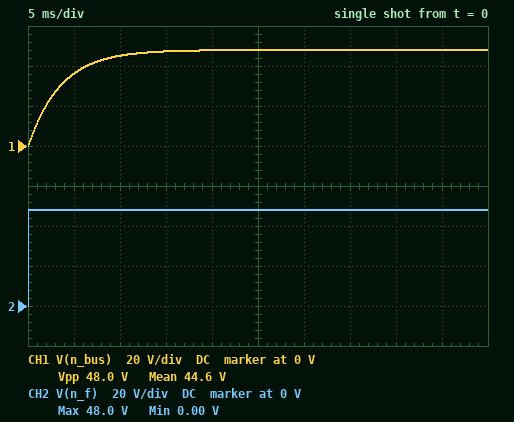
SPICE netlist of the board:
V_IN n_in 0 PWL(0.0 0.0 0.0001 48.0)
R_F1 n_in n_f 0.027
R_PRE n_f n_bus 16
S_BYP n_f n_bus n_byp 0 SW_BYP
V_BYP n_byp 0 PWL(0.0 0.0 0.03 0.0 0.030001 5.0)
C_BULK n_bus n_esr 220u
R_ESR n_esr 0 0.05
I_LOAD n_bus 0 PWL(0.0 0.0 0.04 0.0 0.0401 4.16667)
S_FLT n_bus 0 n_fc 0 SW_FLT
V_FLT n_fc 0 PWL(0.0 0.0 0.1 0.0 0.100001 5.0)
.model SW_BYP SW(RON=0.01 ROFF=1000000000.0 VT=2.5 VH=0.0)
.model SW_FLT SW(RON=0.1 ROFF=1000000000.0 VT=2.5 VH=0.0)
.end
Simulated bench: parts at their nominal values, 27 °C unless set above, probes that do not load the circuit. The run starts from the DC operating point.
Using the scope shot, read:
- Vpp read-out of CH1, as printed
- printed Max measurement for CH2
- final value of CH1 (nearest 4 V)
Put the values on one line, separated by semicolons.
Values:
48.0 V; 48.0 V; 48 V
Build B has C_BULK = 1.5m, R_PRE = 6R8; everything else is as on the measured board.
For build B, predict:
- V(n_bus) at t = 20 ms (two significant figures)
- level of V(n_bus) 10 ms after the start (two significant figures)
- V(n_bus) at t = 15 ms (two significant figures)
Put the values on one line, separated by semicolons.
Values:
41 V; 30 V; 37 V
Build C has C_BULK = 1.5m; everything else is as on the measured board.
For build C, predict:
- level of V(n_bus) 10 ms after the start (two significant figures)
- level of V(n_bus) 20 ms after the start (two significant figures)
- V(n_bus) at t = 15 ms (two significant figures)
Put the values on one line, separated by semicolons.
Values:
16 V; 27 V; 22 V
